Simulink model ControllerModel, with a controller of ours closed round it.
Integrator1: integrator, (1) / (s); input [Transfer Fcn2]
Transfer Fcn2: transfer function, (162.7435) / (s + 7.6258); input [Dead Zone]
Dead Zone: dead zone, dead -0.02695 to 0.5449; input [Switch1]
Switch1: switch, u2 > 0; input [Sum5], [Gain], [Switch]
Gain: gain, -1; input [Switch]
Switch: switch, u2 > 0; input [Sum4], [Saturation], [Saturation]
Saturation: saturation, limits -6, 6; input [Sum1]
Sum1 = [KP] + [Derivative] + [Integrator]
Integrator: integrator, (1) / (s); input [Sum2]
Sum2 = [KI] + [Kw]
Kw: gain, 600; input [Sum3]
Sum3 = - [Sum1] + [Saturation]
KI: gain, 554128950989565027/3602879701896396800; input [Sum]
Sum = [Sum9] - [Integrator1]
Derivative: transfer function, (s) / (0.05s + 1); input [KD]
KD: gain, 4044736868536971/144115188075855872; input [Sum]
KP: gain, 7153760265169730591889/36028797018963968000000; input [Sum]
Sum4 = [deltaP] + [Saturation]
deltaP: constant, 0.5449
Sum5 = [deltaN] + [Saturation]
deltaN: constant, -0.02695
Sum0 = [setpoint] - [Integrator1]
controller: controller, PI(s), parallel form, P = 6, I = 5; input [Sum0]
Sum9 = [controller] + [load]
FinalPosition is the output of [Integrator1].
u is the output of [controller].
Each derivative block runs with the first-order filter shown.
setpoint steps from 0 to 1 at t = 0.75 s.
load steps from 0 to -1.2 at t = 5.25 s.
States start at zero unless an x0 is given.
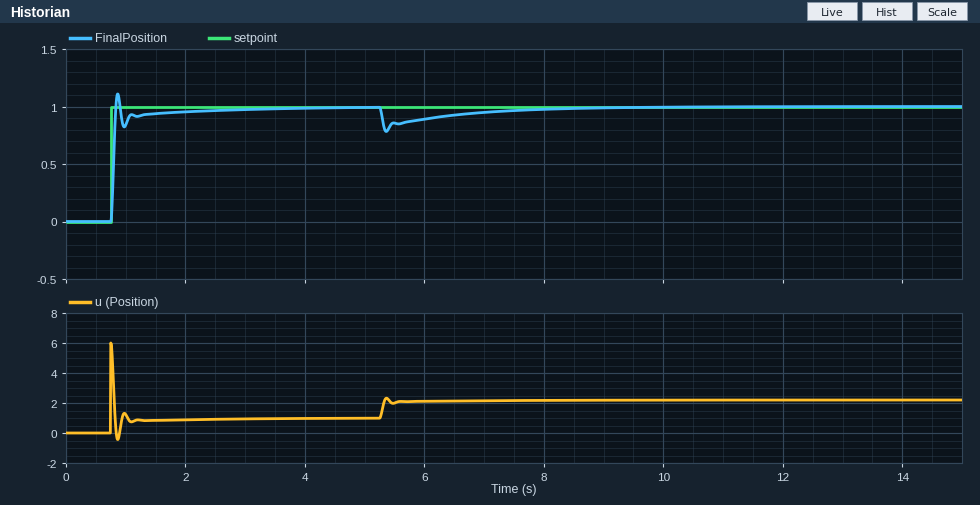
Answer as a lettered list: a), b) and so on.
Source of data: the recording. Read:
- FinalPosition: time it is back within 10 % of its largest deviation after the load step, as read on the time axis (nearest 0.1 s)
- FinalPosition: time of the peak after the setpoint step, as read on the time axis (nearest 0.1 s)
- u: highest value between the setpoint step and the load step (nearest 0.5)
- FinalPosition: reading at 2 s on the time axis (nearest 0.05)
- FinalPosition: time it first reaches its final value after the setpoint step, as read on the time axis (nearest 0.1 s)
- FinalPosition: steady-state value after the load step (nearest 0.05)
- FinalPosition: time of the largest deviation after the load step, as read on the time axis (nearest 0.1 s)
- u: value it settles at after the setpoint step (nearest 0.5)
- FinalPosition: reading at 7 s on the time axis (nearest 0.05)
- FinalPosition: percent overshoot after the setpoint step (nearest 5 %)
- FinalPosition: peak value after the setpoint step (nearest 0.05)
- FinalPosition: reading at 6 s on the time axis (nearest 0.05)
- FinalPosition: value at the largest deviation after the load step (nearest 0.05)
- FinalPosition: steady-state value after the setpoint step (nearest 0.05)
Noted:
a) 8.2 s
b) 0.9 s
c) 6.0
d) 0.95
e) 0.8 s
f) 1.00
g) 5.4 s
h) 1.0
i) 0.95
j) 10 %
k) 1.10
l) 0.90
m) 0.80
n) 1.00
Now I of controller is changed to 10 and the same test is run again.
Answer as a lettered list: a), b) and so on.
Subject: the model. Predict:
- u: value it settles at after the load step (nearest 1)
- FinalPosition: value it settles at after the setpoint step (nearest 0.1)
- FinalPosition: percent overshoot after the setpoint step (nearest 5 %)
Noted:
a) 2
b) 1.0
c) 15 %
